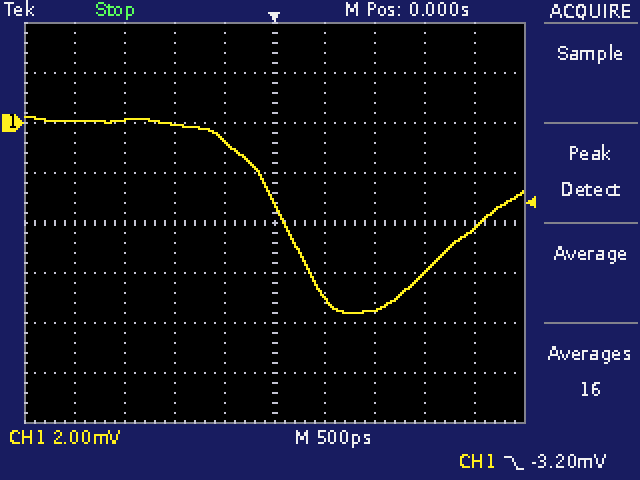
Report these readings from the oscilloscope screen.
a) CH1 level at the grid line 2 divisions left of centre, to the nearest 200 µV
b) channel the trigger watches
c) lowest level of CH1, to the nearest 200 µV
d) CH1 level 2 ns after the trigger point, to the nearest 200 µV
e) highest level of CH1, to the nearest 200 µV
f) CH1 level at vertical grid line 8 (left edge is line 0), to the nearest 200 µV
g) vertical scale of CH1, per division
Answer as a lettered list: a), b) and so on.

a) 0.0 mV
b) CH1
c) -7.6 mV
d) -4.2 mV
e) 200 µV
f) -6.0 mV
g) 2 mV
